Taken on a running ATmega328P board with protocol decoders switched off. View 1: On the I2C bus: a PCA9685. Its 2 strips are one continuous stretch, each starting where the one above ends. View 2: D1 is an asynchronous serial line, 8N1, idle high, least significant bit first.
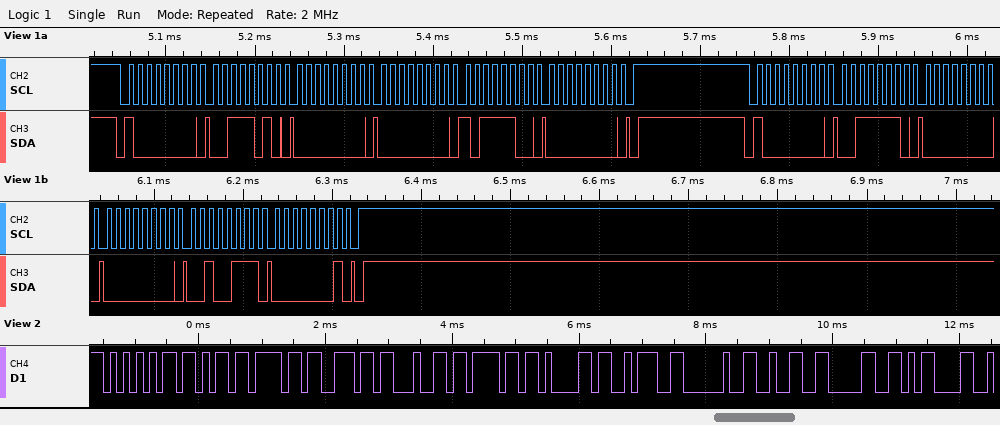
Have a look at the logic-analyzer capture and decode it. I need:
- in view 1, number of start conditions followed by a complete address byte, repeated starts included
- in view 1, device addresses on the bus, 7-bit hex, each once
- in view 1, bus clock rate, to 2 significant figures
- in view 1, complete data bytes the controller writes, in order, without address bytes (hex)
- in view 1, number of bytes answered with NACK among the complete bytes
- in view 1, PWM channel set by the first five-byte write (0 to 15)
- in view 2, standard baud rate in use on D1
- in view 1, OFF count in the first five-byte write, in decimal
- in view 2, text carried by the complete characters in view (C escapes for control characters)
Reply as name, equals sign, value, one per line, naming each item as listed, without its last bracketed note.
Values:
in view 1, number of start conditions followed by a complete address byte, repeated starts included = 2
in view 1, device addresses on the bus, 7-bit hex, each once = 0x40
in view 1, bus clock rate, to 2 significant figures = 100 kHz
in view 1, complete data bytes the controller writes, in order, without address bytes = 3A 00 00 BC 00 3E 00 00 27 01
in view 1, number of bytes answered with NACK among the complete bytes = 0
in view 1, PWM channel set by the first five-byte write = 13
in view 2, standard baud rate in use on D1 = 9600 baud
in view 1, OFF count in the first five-byte write, in decimal = 188
in view 2, text carried by the complete characters in view = "Ukondoa: 20\r"
